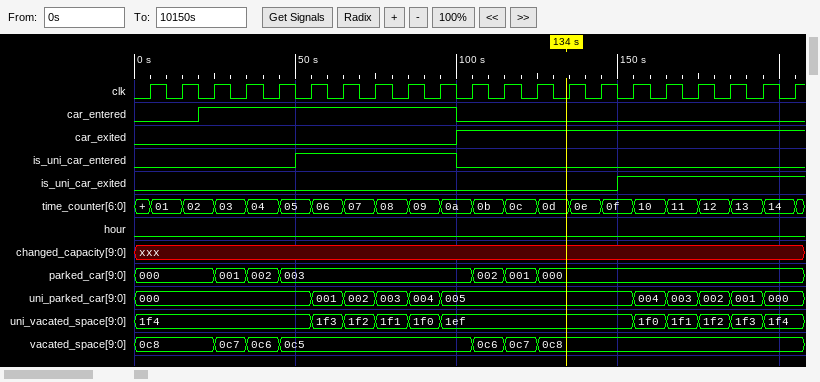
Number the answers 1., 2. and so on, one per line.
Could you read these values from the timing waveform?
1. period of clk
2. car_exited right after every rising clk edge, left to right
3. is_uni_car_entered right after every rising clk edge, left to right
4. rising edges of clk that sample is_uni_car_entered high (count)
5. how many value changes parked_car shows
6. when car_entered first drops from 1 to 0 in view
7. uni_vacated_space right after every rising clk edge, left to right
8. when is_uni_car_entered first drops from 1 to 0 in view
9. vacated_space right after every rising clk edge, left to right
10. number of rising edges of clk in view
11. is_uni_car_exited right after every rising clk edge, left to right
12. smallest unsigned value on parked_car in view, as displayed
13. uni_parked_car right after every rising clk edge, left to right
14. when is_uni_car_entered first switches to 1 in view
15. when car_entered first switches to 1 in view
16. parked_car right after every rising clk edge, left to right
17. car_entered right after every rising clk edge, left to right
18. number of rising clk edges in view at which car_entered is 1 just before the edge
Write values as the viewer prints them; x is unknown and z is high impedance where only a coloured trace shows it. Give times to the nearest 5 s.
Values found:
1. 10 s
2. 0 0 0 0 0 0 0 0 0 0 1 1 1 1 1 1 1 1 1 1 1
3. 0 0 0 0 0 1 1 1 1 1 0 0 0 0 0 0 0 0 0 0 0
4. 5
5. 6
6. 100 s
7. 1f4, 1f4, 1f4, 1f4, 1f4, 1f3, 1f2, 1f1, 1f0, 1ef, 1ef, 1ef, 1ef, 1ef, 1ef, 1f0, 1f1, 1f2, 1f3, 1f4, 1f4
8. 100 s
9. 0c8, 0c8, 0c7, 0c6, 0c5, 0c5, 0c5, 0c5, 0c5, 0c5, 0c6, 0c7, 0c8, 0c8, 0c8, 0c8, 0c8, 0c8, 0c8, 0c8, 0c8
10. 21
11. 0 0 0 0 0 0 0 0 0 0 0 0 0 0 0 1 1 1 1 1 1
12. 000
13. 000, 000, 000, 000, 000, 001, 002, 003, 004, 005, 005, 005, 005, 005, 005, 004, 003, 002, 001, 000, 000
14. 50 s
15. 20 s
16. 000, 000, 001, 002, 003, 003, 003, 003, 003, 003, 002, 001, 000, 000, 000, 000, 000, 000, 000, 000, 000
17. 0 0 1 1 1 1 1 1 1 1 0 0 0 0 0 0 0 0 0 0 0
18. 8
